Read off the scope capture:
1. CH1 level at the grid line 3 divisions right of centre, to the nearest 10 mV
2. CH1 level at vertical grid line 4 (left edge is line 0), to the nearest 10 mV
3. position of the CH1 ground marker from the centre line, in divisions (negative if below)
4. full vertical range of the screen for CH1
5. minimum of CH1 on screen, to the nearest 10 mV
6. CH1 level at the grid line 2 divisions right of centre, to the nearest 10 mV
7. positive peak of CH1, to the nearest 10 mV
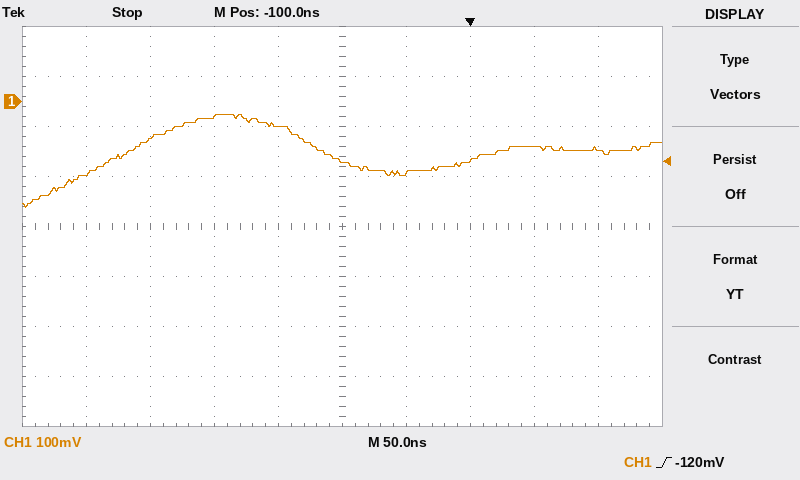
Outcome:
-90 mV
-50 mV
+2.5 div
800 mV
-210 mV
-120 mV
-30 mV
